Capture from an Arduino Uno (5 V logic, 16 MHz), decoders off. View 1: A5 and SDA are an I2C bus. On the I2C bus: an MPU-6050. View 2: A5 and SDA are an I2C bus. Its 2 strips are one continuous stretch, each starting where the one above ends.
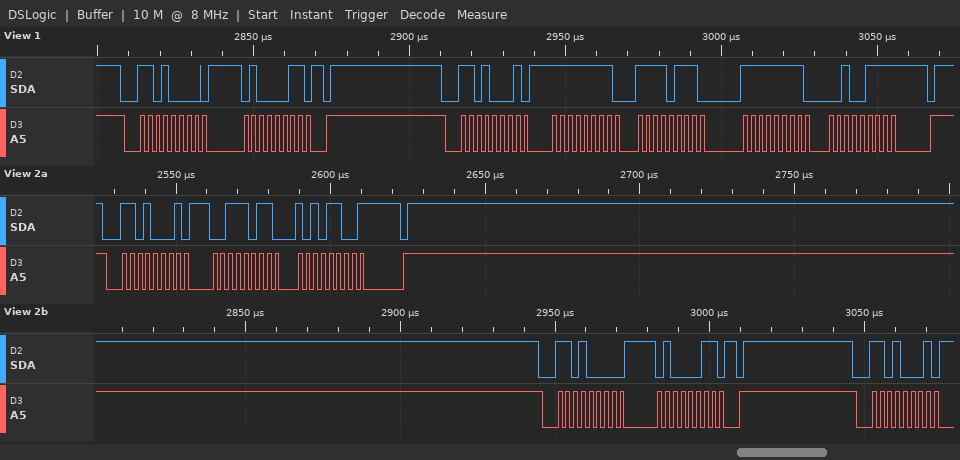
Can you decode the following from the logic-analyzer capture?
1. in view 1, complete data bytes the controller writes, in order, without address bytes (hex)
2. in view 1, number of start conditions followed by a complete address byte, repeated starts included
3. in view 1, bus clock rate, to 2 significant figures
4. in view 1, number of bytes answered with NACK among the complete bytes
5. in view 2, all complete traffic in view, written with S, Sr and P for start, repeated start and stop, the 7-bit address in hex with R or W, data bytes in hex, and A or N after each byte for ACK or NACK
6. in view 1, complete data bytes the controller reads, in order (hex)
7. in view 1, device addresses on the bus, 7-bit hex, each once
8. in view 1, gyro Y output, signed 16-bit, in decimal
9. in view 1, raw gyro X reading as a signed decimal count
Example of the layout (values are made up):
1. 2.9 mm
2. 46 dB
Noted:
1. 43
2. 2
3. 400 kHz
4. 1
5. S 68R A 3B A AC N P S 68W A 43 A P S 68R A
6. FF F7 FF 27
7. 0x68
8. -217
9. -9
